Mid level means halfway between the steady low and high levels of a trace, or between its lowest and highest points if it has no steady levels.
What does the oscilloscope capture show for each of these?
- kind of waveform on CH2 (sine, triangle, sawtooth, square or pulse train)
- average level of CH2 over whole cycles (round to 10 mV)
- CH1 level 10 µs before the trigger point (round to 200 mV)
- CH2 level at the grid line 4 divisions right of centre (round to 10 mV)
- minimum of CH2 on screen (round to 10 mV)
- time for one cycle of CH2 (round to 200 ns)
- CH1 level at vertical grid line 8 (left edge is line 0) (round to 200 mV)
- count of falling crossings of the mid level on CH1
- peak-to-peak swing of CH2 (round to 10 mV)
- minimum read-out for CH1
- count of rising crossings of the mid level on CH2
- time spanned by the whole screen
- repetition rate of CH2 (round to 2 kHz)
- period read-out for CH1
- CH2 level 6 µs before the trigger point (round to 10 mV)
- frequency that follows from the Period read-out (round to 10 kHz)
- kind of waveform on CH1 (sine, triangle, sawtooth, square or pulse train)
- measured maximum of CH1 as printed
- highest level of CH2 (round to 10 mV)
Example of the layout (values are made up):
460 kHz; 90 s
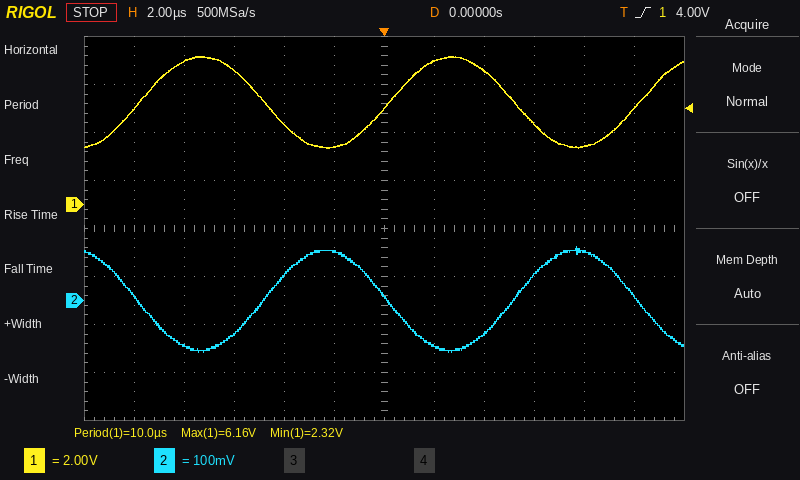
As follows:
sine; 0 mV; 4.0 V; 100 mV; -110 mV; 10.0 µs; 5.6 V; 2; 220 mV; 2.32 V; 2; 24 µs; 100 kHz; 10.0 µs; -70 mV; 100 kHz; sine; 6.16 V; 110 mV
